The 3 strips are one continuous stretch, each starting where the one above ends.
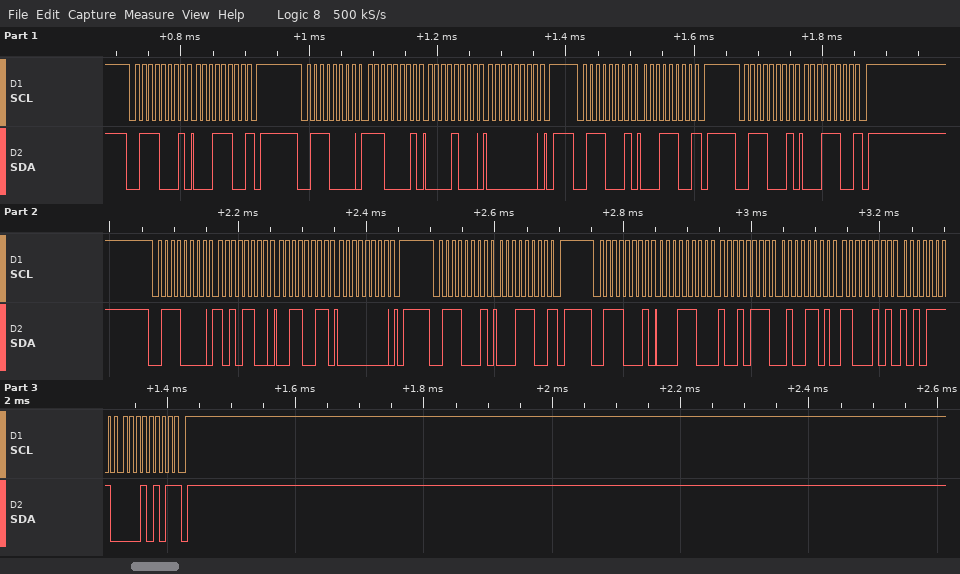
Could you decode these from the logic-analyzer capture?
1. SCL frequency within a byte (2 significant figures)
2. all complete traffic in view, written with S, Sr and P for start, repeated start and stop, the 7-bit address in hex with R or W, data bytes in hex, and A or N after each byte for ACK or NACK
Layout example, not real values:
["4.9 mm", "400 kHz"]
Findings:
["100 kHz", "S 38R A 1C N P S 38W A E1 A 08 A 00 A P S 38R A 1C N P S 38R A 1C N P S 38W A AC A 33 A 00 A P S 38R A 1C N P S 38R A 1C A 97 A 4D A C5 A AF A 15 N P"]
